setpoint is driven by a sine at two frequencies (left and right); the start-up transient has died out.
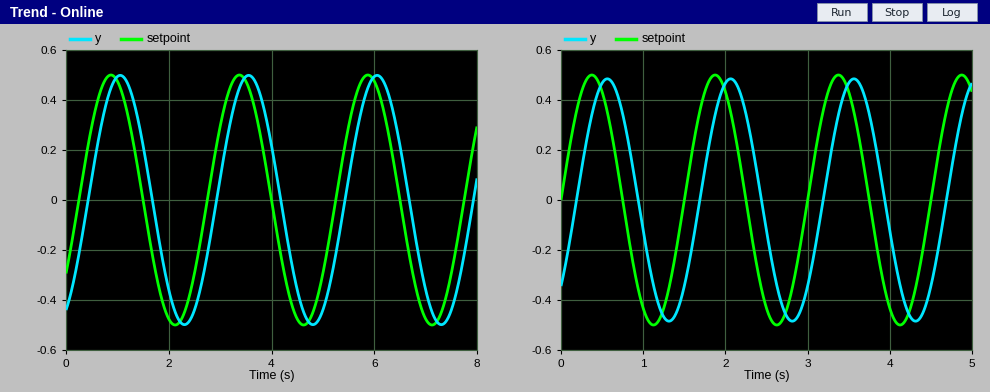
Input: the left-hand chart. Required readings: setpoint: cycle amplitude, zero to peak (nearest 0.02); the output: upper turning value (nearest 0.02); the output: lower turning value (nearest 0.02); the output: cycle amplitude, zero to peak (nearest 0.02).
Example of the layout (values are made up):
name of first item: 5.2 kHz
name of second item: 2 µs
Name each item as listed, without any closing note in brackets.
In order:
setpoint: cycle amplitude, zero to peak: 0.50
the output: upper turning value: 0.50
the output: lower turning value: -0.50
the output: cycle amplitude, zero to peak: 0.50
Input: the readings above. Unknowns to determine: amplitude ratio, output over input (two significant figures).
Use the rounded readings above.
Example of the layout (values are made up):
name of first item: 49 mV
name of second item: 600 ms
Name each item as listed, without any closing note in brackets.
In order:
amplitude ratio, output over input: 1.0
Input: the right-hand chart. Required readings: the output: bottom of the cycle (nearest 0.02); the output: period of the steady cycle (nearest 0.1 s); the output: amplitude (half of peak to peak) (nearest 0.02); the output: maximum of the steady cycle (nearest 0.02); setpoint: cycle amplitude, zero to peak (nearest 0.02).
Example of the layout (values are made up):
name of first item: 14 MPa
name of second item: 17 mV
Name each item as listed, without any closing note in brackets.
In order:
the output: bottom of the cycle: -0.48
the output: period of the steady cycle: 1.5 s
the output: amplitude (half of peak to peak): 0.48
the output: maximum of the steady cycle: 0.48
setpoint: cycle amplitude, zero to peak: 0.50
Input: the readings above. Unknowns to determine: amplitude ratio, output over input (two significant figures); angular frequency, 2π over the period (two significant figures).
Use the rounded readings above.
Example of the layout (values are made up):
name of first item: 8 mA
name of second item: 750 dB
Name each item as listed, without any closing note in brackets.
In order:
amplitude ratio, output over input: 0.96
angular frequency, 2π over the period: 4.2 rad/s
